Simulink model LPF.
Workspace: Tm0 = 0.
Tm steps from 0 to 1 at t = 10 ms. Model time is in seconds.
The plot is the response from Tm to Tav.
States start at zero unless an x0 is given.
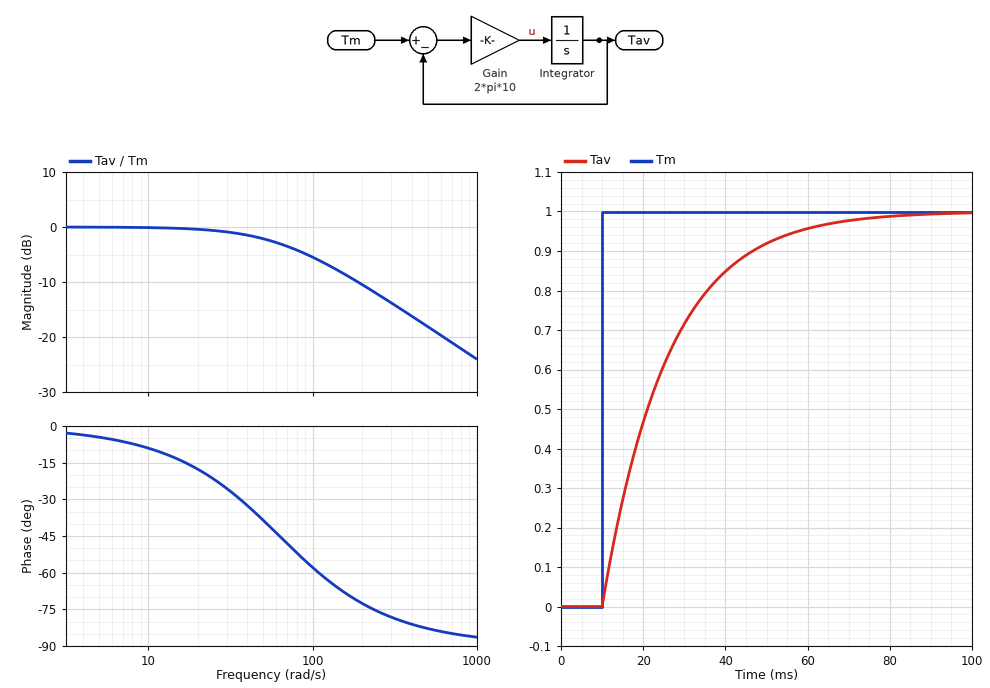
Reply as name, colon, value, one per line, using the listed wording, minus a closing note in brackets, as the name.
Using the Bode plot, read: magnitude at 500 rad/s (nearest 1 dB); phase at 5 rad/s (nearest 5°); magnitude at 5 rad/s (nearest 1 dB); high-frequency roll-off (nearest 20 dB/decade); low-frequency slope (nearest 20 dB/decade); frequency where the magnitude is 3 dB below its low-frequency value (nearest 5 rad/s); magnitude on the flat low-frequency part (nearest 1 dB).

magnitude at 500 rad/s: -18 dB
phase at 5 rad/s: -5°
magnitude at 5 rad/s: 0 dB
high-frequency roll-off: -20 dB/decade
low-frequency slope: 0 dB/decade
frequency where the magnitude is 3 dB below its low-frequency value: 65 rad/s
magnitude on the flat low-frequency part: 0 dB
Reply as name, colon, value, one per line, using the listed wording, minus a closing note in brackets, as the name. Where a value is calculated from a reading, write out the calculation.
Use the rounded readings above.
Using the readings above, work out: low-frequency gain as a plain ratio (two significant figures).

low-frequency gain as a plain ratio: 10^(0 / 20) = 1.0
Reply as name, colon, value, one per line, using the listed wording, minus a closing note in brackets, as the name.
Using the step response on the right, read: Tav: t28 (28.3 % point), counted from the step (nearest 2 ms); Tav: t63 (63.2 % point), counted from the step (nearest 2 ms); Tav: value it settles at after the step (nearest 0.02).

Tav: t28 (28.3 % point), counted from the step: 6 ms
Tav: t63 (63.2 % point), counted from the step: 16 ms
Tav: value it settles at after the step: 1.00
